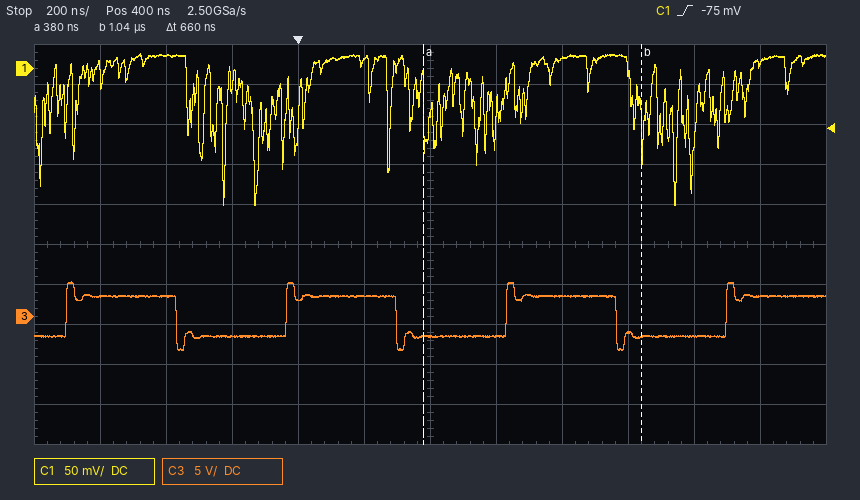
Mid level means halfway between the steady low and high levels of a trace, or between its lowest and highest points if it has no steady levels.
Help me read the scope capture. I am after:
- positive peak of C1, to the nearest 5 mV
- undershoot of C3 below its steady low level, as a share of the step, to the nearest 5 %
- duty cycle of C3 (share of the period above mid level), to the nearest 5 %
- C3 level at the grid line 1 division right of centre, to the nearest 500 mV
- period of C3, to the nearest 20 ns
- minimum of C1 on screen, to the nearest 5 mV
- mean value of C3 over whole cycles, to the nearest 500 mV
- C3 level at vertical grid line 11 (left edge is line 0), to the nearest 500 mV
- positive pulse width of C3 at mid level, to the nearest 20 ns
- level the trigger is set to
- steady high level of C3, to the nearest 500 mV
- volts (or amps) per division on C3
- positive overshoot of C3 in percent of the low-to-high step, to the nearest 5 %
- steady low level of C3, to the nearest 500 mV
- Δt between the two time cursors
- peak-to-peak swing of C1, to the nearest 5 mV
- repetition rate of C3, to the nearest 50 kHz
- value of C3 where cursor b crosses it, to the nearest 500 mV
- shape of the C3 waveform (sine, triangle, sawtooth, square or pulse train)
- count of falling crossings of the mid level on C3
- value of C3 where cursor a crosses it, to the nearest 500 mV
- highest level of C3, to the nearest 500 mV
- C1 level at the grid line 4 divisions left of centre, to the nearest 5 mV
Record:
20 mV
35 %
50 %
-2.5 V
660 ns
-170 mV
0.0 V
2.5 V
340 ns
-75 mV
2.5 V
5 V
35 %
-2.5 V
660 ns
190 mV
1.50 MHz
-2.5 V
square
3
-2.5 V
4.5 V
15 mV
